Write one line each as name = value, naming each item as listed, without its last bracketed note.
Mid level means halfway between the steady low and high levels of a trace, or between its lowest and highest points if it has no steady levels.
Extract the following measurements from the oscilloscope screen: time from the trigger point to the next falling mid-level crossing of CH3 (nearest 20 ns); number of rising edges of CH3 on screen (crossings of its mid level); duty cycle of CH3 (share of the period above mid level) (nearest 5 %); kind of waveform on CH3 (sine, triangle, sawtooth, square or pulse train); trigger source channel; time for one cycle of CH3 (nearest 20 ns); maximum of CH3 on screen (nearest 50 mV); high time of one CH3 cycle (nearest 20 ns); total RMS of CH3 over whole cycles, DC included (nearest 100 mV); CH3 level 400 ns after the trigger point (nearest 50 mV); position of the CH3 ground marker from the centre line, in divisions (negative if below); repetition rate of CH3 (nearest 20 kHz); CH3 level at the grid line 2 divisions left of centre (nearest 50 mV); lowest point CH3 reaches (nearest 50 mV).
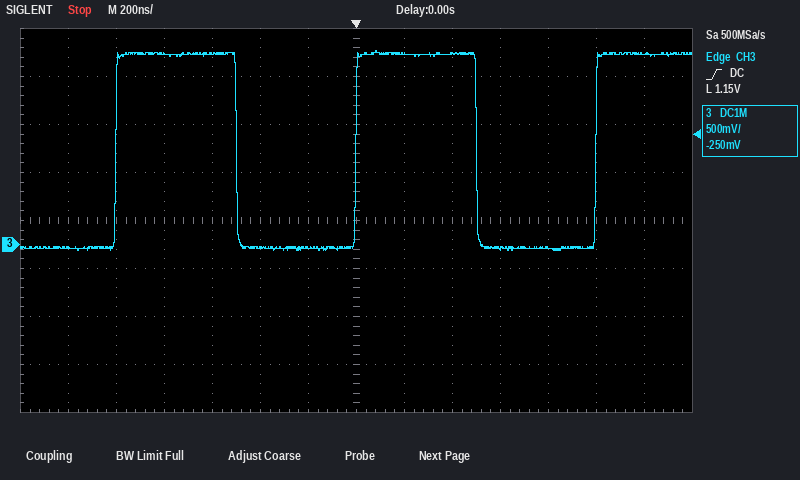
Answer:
time from the trigger point to the next falling mid-level crossing of CH3 = 500 ns
number of rising edges of CH3 on screen = 3
duty cycle of CH3 (share of the period above mid level) = 50 %
kind of waveform on CH3 = square
trigger source channel = CH3
time for one cycle of CH3 = 1.00 µs
maximum of CH3 on screen = 2.00 V
high time of one CH3 cycle = 500 ns
total RMS of CH3 over whole cycles, DC included = 1.4 V
CH3 level 400 ns after the trigger point = 2.00 V
position of the CH3 ground marker from the centre line, in divisions = -0.5 div
repetition rate of CH3 = 1.00 MHz
CH3 level at the grid line 2 divisions left of centre = -50 mV
lowest point CH3 reaches = -50 mV
